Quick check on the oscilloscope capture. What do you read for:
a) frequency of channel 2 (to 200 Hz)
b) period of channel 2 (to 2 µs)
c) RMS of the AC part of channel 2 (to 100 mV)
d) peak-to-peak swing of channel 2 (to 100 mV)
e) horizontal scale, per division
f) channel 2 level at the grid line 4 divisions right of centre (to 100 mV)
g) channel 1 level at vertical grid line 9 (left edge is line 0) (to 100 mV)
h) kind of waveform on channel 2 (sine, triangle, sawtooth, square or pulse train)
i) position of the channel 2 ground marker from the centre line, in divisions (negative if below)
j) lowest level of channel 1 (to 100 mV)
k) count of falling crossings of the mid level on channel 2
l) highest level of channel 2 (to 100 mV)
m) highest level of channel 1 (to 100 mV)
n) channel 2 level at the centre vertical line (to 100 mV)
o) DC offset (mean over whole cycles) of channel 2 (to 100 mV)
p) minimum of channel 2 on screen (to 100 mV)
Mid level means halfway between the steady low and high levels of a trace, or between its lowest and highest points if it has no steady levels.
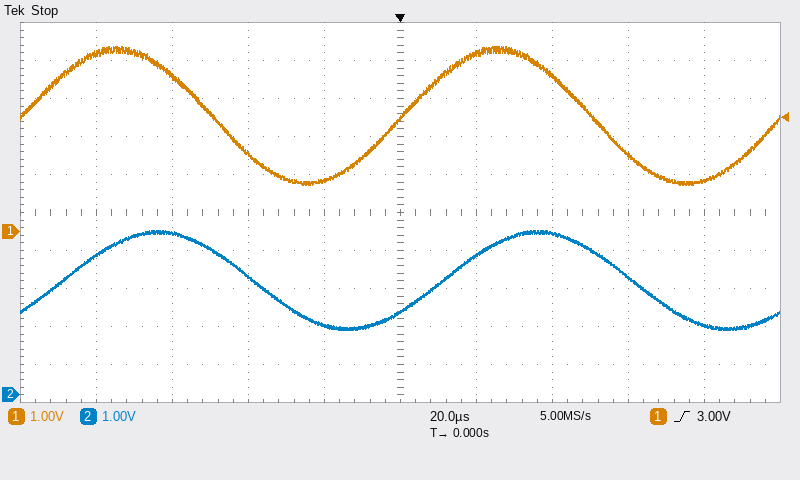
10.0 kHz
100 µs
900 mV
2.6 V
20 µs
1.8 V
1.3 V
sine
-4.8 div
1.2 V
2
4.3 V
4.9 V
2.2 V
3.0 V
1.7 V
